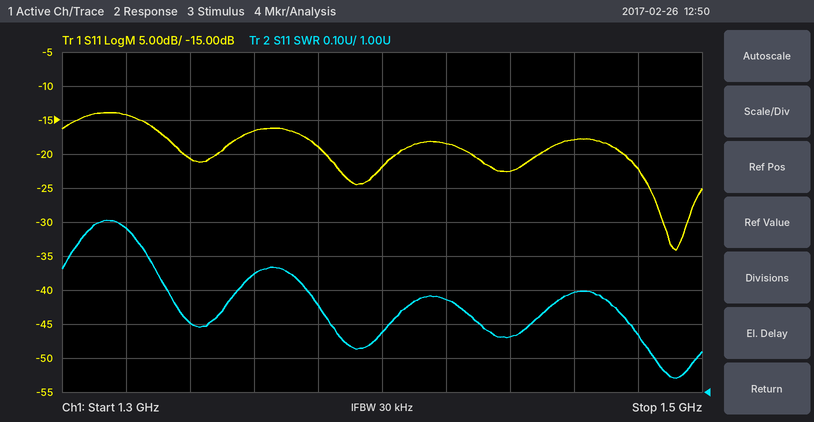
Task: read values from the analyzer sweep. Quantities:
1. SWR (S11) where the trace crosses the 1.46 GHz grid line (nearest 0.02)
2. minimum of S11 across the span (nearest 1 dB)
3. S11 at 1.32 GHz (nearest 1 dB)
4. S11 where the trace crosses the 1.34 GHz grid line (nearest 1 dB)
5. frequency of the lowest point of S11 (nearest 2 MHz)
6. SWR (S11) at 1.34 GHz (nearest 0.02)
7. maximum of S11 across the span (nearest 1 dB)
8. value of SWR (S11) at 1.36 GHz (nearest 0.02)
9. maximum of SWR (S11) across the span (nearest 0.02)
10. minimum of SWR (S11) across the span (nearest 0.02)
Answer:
1.30
-34 dB
-14 dB
-21 dB
1.492 GHz
1.20
-14 dB
1.34
1.50
1.04
